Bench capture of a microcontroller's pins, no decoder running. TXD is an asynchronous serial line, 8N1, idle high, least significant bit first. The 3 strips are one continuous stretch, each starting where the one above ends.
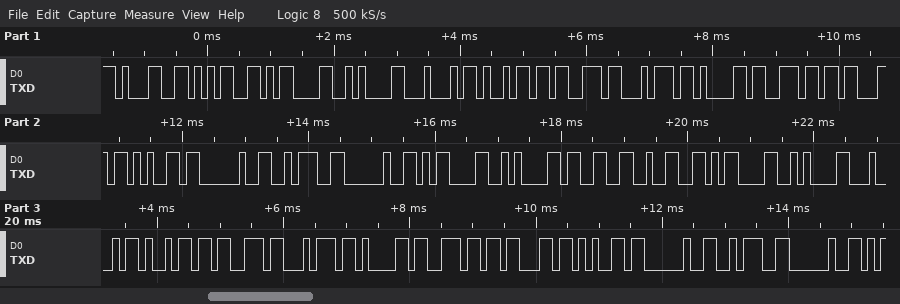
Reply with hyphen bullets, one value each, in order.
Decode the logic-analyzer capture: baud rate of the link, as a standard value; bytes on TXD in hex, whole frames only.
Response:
- 9600 baud
- 31 35 0D 0A 44 69 73 74 61 6E 63 65 20 3A 20 0D 0A 33 32 0D 0A 44 69 73 74 61 6E 63 65 20 3A 20
